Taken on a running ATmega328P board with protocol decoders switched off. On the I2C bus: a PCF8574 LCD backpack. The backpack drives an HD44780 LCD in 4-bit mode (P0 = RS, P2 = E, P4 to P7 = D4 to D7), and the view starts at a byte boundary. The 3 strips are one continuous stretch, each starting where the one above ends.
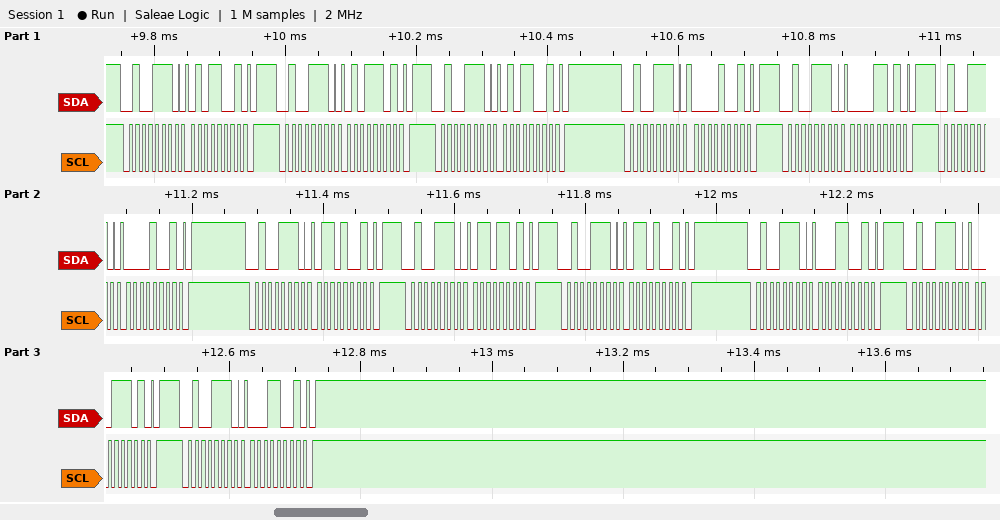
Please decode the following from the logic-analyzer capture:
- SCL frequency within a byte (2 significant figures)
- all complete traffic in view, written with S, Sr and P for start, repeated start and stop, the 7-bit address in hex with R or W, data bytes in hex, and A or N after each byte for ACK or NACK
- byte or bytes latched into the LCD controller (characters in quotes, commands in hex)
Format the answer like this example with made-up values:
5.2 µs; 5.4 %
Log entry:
100 kHz; S 27W A 59 A P S 27W A 5D A P S 27W A 59 A P S 27W A 09 A P S 27W A 0D A P S 27W A 09 A P S 27W A 69 A P S 27W A 6D A P S 27W A 69 A P S 27W A 19 A P S 27W A 1D A P S 27W A 19 A P; 'P' 'a'
